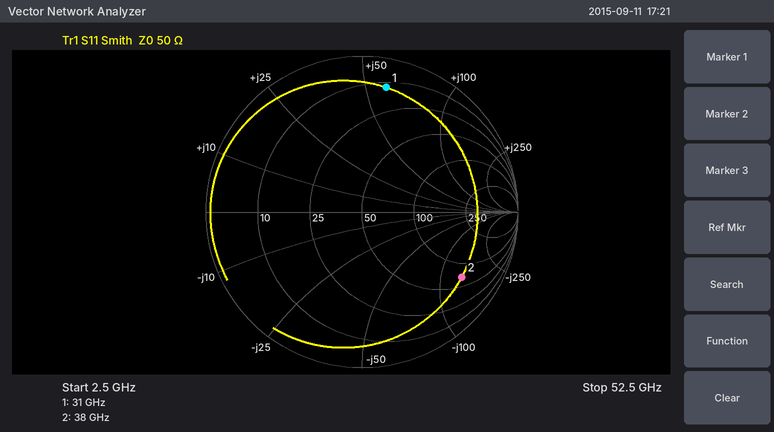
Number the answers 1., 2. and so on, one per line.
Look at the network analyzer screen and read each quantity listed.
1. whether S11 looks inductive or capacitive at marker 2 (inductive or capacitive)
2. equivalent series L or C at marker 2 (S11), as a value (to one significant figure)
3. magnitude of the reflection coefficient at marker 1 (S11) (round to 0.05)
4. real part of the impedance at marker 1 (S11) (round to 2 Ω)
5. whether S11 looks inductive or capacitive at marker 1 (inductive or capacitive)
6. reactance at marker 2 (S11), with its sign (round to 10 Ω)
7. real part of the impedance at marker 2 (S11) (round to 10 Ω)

1. capacitive
2. 30 fF
3. 0.80
4. 12 Ω
5. inductive
6. -140 Ω
7. 70 Ω
